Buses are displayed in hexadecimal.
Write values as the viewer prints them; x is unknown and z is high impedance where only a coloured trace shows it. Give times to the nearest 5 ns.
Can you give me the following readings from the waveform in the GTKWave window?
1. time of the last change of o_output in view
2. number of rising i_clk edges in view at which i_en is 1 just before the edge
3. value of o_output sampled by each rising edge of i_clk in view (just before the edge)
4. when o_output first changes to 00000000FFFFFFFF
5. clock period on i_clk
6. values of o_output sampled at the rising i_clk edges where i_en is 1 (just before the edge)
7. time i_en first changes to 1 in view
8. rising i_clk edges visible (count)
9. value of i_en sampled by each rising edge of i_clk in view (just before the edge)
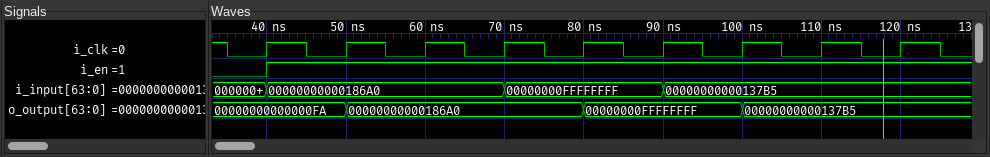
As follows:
100 ns
8
00000000000000FA, 00000000000000FA, 00000000000186A0, 00000000000186A0, 00000000000186A0, 00000000FFFFFFFF, 00000000FFFFFFFF, 00000000000137B5, 00000000000137B5
80 ns
10 ns
00000000000000FA, 00000000000186A0, 00000000000186A0, 00000000000186A0, 00000000FFFFFFFF, 00000000FFFFFFFF, 00000000000137B5, 00000000000137B5
40 ns
9
0 1 1 1 1 1 1 1 1
